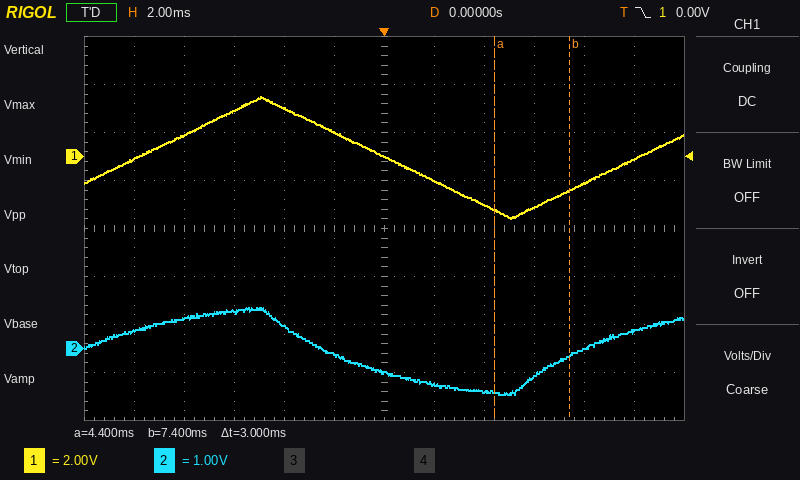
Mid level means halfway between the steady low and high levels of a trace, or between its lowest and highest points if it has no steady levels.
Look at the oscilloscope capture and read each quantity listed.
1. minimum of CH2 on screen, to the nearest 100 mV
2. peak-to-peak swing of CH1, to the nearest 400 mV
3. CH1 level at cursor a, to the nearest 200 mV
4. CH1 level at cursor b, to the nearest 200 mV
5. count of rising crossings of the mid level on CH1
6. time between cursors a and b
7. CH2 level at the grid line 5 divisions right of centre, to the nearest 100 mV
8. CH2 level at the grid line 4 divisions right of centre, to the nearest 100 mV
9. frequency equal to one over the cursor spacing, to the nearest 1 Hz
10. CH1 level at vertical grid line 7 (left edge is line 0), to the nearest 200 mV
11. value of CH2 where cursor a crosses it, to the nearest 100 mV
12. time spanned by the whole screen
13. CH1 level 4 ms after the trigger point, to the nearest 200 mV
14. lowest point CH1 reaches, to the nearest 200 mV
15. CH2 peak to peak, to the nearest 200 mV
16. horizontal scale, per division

-1.0 V
5.2 V
-2.2 V
-1.4 V
2
3 ms
400 mV
0.0 V
333 Hz
-1.0 V
-900 mV
24 ms
-2.0 V
-2.6 V
1.8 V
2 ms
